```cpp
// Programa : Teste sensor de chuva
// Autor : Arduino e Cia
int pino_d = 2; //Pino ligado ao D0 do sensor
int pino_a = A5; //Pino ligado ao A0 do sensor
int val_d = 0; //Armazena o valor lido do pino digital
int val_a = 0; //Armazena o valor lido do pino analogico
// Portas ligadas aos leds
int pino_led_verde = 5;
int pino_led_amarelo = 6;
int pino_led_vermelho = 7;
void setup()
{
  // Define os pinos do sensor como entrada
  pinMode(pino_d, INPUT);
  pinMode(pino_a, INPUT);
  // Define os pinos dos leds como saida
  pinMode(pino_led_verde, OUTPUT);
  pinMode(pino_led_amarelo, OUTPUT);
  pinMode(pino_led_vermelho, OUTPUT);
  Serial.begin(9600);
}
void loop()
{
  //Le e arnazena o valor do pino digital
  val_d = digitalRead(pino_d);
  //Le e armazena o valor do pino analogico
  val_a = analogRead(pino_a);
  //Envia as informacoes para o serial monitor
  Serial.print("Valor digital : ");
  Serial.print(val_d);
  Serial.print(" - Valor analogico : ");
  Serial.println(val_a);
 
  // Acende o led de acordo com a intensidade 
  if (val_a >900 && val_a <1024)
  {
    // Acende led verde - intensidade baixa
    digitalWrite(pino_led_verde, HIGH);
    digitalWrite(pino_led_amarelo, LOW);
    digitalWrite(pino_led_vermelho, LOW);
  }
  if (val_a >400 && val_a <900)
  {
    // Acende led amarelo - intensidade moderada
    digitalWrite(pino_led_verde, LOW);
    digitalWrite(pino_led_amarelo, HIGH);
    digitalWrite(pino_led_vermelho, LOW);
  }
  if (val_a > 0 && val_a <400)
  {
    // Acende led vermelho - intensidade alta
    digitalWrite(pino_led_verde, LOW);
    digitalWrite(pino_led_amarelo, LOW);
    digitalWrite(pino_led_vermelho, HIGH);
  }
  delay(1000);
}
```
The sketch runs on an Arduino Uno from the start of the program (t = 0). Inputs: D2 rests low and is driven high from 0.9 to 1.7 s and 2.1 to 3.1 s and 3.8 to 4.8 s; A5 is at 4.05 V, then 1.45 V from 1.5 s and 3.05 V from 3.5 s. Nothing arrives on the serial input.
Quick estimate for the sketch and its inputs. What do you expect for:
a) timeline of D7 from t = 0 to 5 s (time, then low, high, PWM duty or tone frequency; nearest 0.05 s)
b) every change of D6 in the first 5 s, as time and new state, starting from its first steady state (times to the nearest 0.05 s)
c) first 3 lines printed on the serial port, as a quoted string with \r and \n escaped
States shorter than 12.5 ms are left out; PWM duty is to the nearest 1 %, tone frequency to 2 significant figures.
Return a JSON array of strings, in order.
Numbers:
["0 s low; 2 s high; 4 s low", "0 s high; 2 s low; 4 s high", "\"Valor digital : 0 - Valor analogico : 829\\r\\nValor digital : 1 - Valor analogico : 829\\r\\nValor digital : 0 - Valor analogico : 296\\r\\n\""]
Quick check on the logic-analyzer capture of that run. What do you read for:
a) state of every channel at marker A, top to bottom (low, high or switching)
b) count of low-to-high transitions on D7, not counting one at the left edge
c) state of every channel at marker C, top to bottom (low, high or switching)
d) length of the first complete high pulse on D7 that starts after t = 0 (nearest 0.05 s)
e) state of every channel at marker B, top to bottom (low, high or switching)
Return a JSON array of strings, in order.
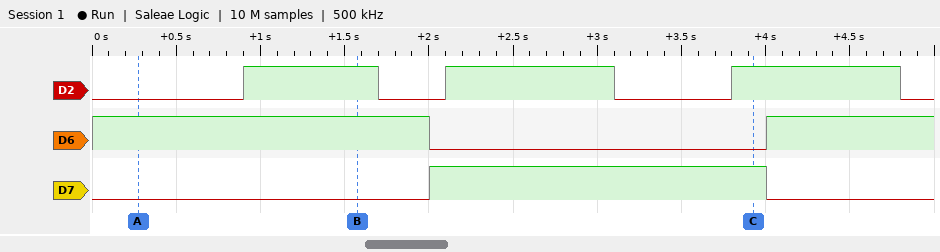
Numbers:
["D2 low, D6 high, D7 low", "1", "D2 high, D6 low, D7 high", "2.00 s", "D2 high, D6 high, D7 low"]
